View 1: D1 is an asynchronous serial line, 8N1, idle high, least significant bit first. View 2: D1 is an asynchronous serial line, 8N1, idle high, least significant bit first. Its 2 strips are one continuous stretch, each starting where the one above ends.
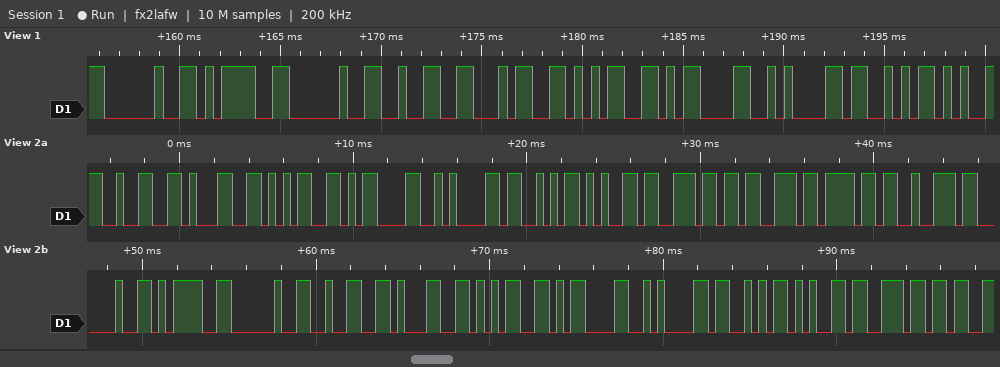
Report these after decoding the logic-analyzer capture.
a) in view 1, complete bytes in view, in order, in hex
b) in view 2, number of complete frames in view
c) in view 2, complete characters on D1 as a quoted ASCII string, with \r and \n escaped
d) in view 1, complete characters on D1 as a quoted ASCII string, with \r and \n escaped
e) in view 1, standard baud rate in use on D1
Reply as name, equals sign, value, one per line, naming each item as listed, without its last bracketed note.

in view 1, complete bytes in view, in order, in hex = 20 3D 20 32 34 35 0D 0A 53
in view 2, number of complete frames in view = 22
in view 2, complete characters on D1 as a quoted ASCII string, with \r and \n escaped = "215\r\nSensor = 215\r\nSen"
in view 1, complete characters on D1 as a quoted ASCII string, with \r and \n escaped = " = 245\r\nS"
in view 1, standard baud rate in use on D1 = 2400 baud
